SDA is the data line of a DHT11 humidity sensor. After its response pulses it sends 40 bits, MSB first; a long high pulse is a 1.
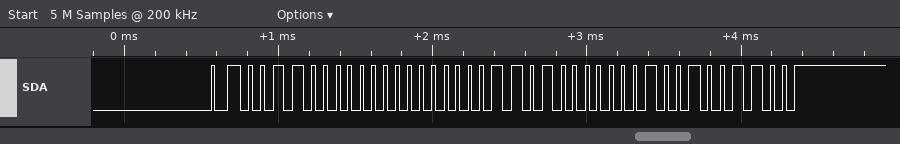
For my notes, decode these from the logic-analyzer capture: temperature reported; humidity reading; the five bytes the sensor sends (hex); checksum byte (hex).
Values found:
26.2 °C
48 %
30 00 1A 02 4C
0x4C
